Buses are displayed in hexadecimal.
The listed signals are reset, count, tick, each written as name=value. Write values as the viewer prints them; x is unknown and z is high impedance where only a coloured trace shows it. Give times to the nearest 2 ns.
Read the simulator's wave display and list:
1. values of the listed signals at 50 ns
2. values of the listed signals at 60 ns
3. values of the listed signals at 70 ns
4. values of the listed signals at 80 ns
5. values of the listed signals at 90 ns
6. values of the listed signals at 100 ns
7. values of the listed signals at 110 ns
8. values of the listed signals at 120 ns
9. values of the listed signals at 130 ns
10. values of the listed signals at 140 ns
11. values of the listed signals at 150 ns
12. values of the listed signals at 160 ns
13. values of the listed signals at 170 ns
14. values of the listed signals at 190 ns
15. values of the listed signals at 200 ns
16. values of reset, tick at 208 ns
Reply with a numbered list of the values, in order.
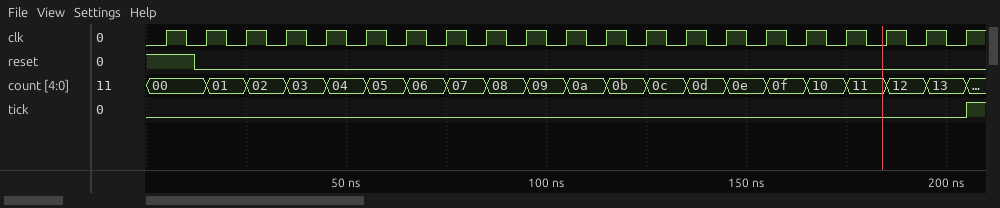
1. reset=0, count=04, tick=0
2. reset=0, count=05, tick=0
3. reset=0, count=06, tick=0
4. reset=0, count=07, tick=0
5. reset=0, count=08, tick=0
6. reset=0, count=09, tick=0
7. reset=0, count=0a, tick=0
8. reset=0, count=0b, tick=0
9. reset=0, count=0c, tick=0
10. reset=0, count=0d, tick=0
11. reset=0, count=0e, tick=0
12. reset=0, count=0f, tick=0
13. reset=0, count=10, tick=0
14. reset=0, count=12, tick=0
15. reset=0, count=13, tick=0
16. reset=0, tick=1
